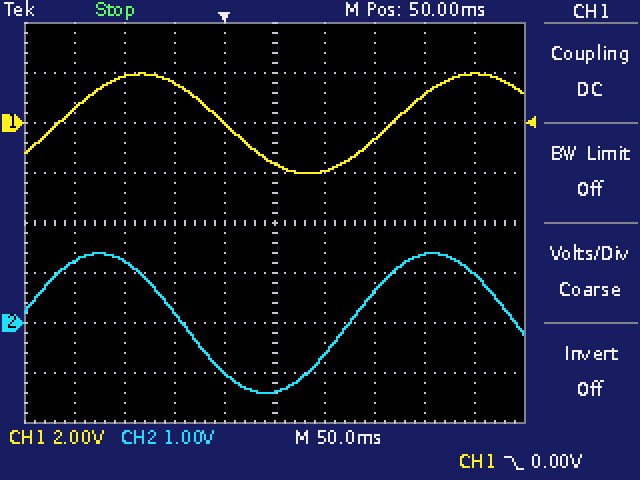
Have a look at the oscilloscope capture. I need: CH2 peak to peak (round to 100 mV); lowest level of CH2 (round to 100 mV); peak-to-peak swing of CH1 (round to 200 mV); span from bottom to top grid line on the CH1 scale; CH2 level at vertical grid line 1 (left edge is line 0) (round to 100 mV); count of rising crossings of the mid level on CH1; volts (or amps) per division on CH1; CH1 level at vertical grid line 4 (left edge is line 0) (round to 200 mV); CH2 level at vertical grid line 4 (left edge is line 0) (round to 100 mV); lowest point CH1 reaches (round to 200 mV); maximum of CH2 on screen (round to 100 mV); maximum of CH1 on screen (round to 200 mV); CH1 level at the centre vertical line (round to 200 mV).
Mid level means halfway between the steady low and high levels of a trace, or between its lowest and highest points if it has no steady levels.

2.8 V
-1.4 V
4.0 V
16 V
1.2 V
2
2 V
0.0 V
-1.0 V
-2.0 V
1.4 V
2.0 V
-1.6 V
